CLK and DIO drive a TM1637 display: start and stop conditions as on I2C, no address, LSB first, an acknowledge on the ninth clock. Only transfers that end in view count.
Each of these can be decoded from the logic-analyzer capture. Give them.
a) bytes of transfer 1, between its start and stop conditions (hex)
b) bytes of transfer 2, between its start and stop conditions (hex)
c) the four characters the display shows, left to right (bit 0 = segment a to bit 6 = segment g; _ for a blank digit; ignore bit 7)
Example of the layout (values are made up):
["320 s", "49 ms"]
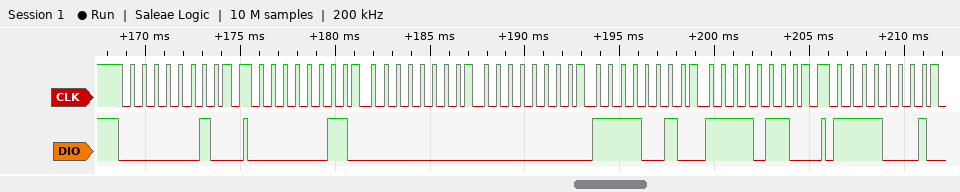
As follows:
["40", "C0 00 00 4F 6F", "__39"]
